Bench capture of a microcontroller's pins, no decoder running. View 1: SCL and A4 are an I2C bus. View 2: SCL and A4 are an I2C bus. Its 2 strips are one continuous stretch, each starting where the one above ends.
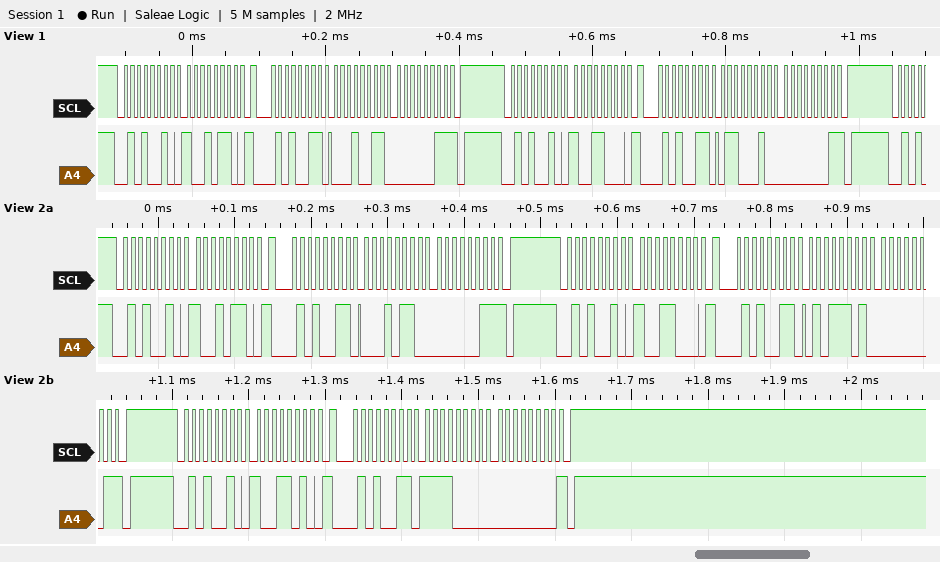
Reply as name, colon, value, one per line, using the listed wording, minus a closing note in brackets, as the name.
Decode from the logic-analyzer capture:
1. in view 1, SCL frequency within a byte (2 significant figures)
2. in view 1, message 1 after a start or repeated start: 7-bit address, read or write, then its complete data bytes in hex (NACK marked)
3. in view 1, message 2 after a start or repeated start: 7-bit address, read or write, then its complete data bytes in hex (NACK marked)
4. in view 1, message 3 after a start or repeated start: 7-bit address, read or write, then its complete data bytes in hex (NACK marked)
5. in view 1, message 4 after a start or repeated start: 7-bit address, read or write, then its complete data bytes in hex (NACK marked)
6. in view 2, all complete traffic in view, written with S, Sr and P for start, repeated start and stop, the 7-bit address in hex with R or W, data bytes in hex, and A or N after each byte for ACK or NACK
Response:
in view 1, SCL frequency within a byte: 100 kHz
in view 1, message 1 after a start or repeated start: 7-bit address, read or write, then its complete data bytes in hex: 0x29 write: 96
in view 1, message 2 after a start or repeated start: 7-bit address, read or write, then its complete data bytes in hex: 0x29 read: 13 03 NACK
in view 1, message 3 after a start or repeated start: 7-bit address, read or write, then its complete data bytes in hex: 0x29 write: 98
in view 1, message 4 after a start or repeated start: 7-bit address, read or write, then its complete data bytes in hex: 0x29 read: 62 01 NACK
in view 2, all complete traffic in view, written with S, Sr and P for start, repeated start and stop, the 7-bit address in hex with R or W, data bytes in hex, and A or N after each byte for ACK or NACK: S 29W A 96 A Sr 29R A 16 A 03 N P S 29W A 98 A Sr 29R A 5D A 01 N P S 29W A 9A A Sr 29R A F0 A 00 N P
